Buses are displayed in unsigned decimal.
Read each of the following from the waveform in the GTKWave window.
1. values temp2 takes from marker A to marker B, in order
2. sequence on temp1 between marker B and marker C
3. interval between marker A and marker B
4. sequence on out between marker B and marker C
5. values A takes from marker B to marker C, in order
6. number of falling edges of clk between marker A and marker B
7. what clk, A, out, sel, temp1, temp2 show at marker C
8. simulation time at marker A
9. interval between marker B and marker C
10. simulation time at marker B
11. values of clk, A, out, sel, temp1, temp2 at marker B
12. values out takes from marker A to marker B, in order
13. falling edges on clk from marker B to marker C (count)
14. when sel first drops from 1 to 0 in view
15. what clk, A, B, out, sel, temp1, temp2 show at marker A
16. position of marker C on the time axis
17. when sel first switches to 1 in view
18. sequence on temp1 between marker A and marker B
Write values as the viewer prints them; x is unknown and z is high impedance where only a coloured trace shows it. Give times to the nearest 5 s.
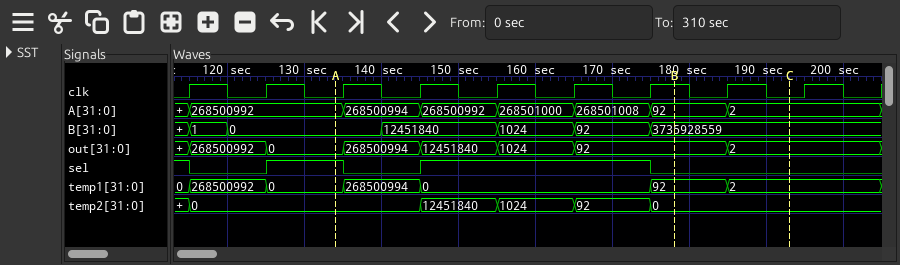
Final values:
0, 12451840, 1024, 92, 0
92, 2
45 s
92, 2
92, 2
4
clk=0, A=2, out=2, sel=0, temp1=2, temp2=0
135 s
15 s
180 s
clk=1, A=92, out=92, sel=0, temp1=92, temp2=0
0, 268500994, 12451840, 1024, 92
2
115 s
clk=0, A=268500992, B=0, out=0, sel=1, temp1=0, temp2=0
195 s
125 s
0, 268500994, 0, 92
